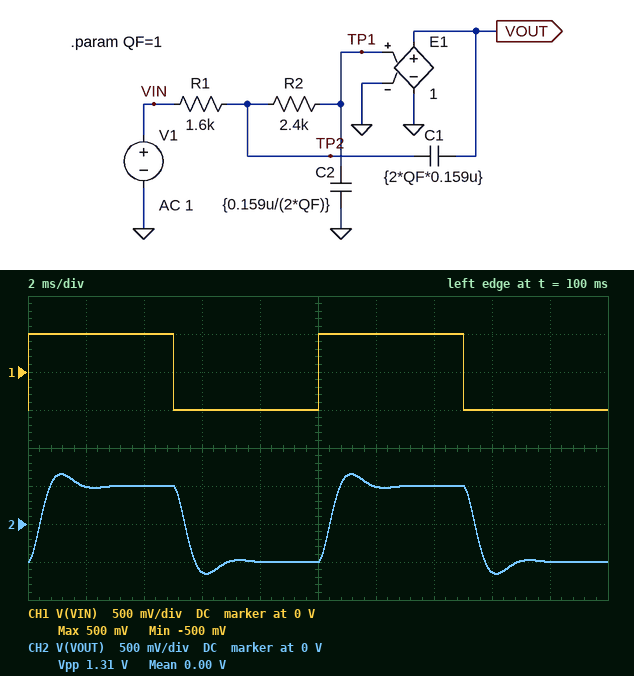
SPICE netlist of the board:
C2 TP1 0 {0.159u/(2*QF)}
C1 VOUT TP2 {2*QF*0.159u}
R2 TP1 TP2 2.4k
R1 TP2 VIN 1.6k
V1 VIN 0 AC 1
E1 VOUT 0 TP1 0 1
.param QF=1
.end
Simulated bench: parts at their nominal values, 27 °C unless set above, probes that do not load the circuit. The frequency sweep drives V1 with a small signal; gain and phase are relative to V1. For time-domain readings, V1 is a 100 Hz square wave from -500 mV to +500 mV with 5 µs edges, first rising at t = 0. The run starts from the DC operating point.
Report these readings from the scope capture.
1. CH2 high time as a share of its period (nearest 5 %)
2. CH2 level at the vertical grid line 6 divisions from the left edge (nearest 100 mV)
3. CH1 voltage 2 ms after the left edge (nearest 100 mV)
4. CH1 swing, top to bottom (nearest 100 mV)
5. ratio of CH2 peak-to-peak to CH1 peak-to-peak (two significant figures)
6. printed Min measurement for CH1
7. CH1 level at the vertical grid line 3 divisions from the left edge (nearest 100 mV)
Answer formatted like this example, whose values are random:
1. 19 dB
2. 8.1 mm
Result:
1. 50 %
2. 500 mV
3. 500 mV
4. 1.0 V
5. 1.3
6. -500 mV
7. -500 mV
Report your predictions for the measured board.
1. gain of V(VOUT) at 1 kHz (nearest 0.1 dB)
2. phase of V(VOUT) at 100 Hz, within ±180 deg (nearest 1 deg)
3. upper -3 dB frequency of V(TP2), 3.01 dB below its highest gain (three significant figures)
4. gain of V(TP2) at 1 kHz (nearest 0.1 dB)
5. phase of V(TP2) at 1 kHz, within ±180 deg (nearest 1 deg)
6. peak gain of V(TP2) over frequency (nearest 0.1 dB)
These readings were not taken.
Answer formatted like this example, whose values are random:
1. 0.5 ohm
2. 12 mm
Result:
1. -10.8 dB
2. -12 deg
3. 649 Hz
4. -6.9 dB
5. -95 deg
6. 1.9 dB
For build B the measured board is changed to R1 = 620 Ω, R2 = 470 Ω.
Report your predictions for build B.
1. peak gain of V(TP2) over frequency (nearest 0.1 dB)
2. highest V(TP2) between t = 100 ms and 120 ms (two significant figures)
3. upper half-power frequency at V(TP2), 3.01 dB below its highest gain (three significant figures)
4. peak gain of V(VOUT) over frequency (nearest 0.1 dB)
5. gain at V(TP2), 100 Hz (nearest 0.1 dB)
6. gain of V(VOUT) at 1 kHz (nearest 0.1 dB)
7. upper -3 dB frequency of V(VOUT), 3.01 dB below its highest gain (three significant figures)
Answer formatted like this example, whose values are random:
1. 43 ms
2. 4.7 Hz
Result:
1. 1.6 dB
2. 680 mV
3. 2.27 kHz
4. 1.2 dB
5. 0 dB
6. 1.0 dB
7. 2.16 kHz
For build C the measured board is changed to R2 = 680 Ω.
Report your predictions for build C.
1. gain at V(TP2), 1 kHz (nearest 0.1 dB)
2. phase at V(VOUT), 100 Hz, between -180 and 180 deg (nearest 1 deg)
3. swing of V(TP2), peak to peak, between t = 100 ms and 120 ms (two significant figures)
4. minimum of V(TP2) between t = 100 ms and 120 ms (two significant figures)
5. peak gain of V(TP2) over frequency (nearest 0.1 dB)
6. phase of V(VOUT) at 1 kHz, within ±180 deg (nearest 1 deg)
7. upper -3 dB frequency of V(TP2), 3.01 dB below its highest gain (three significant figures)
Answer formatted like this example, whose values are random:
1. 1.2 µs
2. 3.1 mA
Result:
1. -0.7 dB
2. -7 deg
3. 1.3 V
4. -640 mV
5. 1.0 dB
6. -94 deg
7. 1.14 kHz
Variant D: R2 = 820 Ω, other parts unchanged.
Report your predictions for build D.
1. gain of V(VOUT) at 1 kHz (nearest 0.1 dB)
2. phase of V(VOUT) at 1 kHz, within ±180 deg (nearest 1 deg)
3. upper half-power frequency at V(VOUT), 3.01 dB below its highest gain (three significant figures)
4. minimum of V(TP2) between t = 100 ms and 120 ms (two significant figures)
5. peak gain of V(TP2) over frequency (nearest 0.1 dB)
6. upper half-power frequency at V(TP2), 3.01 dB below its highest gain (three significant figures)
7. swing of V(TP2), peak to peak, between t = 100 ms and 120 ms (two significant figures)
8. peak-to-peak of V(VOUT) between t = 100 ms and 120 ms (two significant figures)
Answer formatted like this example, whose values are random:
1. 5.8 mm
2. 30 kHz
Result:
1. -1.9 dB
2. -104 deg
3. 1.01 kHz
4. -650 mV
5. 1.2 dB
6. 1.05 kHz
7. 1.3 V
8. 1.3 V
